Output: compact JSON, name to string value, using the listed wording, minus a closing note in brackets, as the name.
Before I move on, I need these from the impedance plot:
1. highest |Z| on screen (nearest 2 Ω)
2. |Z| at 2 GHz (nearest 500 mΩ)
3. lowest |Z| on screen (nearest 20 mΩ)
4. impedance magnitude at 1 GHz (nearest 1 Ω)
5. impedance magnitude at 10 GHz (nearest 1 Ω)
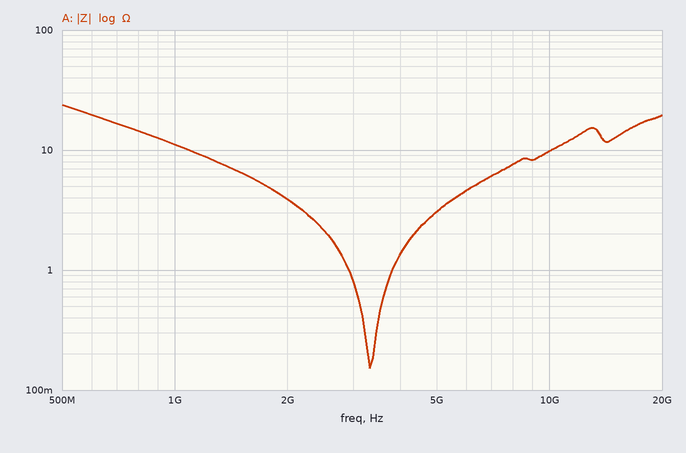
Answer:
{"highest |Z| on screen": "24 Ω", "|Z| at 2 GHz": "4.0 Ω", "lowest |Z| on screen": "160 mΩ", "impedance magnitude at 1 GHz": "11 Ω", "impedance magnitude at 10 GHz": "10 Ω"}
